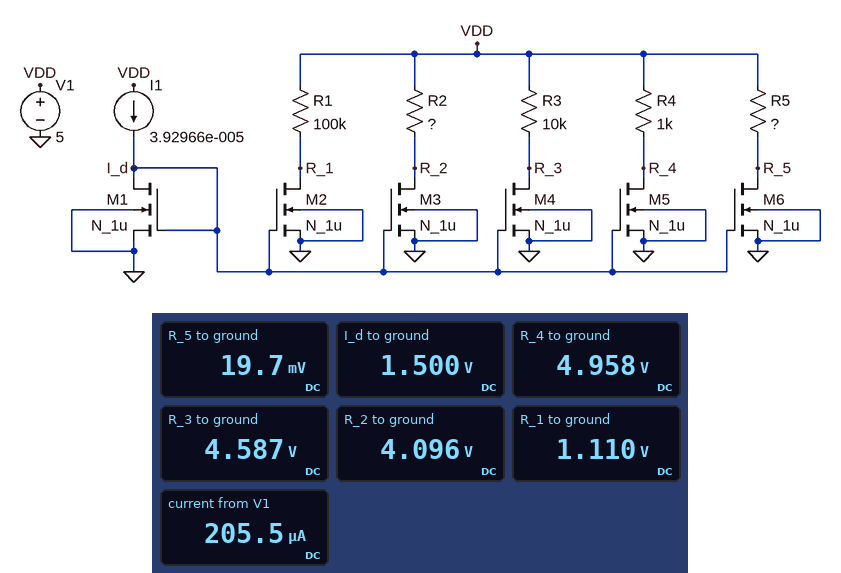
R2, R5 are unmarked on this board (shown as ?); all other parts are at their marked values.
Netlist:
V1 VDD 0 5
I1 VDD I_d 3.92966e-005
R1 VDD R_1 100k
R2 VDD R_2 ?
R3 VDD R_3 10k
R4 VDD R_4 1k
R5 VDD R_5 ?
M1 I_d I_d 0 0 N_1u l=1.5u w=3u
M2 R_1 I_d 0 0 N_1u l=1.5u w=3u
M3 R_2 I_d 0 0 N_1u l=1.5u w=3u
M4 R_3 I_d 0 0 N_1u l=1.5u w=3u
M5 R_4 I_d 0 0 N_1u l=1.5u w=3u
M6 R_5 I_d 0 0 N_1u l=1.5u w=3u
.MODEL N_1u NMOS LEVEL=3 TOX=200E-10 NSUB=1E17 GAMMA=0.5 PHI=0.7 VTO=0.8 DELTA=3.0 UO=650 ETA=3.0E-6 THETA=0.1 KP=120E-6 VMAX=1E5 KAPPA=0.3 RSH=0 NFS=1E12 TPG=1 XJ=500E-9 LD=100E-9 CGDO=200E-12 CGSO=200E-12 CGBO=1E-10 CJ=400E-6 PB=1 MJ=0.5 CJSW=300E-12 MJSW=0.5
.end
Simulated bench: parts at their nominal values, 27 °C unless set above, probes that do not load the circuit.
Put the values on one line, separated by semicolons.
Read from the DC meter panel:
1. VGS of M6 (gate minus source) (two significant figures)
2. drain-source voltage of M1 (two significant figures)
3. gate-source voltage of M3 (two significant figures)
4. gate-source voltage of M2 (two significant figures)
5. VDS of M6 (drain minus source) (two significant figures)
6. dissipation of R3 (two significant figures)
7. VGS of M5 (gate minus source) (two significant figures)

1.5 V; 1.5 V; 1.5 V; 1.5 V; 20 mV; 17 µW; 1.5 V
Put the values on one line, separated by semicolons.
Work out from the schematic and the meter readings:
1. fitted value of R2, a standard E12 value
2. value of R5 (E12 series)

22 kΩ; 1.5 MΩ
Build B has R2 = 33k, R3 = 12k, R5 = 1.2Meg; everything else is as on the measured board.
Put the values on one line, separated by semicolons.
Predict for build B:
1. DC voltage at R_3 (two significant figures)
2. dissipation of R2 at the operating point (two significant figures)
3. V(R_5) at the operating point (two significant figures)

4.5 V; 55 µW; 25 mV
